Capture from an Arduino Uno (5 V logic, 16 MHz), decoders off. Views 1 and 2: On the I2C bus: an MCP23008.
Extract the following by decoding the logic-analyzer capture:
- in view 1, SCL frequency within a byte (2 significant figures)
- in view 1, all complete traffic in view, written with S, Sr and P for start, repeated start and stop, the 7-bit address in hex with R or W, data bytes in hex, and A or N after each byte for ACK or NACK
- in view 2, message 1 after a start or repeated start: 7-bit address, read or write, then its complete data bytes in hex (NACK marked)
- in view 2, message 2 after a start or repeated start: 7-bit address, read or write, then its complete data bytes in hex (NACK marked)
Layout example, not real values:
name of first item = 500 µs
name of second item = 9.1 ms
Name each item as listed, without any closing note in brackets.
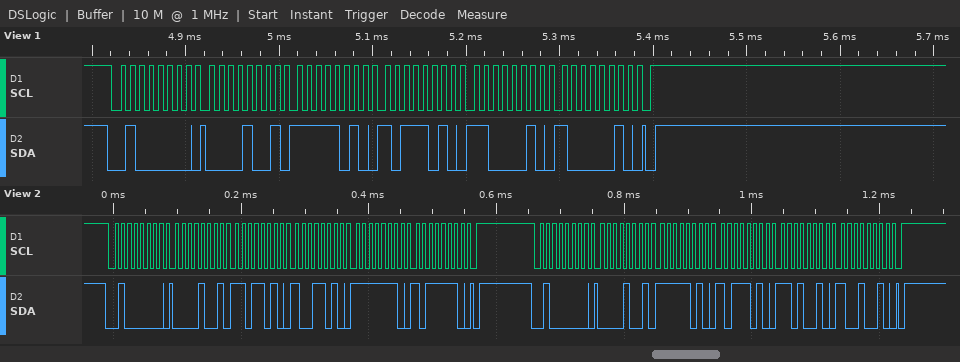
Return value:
in view 1, SCL frequency within a byte = 100 kHz
in view 1, all complete traffic in view, written with S, Sr and P for start, repeated start and stop, the 7-bit address in hex with R or W, data bytes in hex, and A or N after each byte for ACK or NACK = S 20W A 09 A FA A BA A C2 A 82 A P
in view 2, message 1 after a start or repeated start: 7-bit address, read or write, then its complete data bytes in hex = 0x20 write: 09 DA 9A FE BE
in view 2, message 2 after a start or repeated start: 7-bit address, read or write, then its complete data bytes in hex = 0x20 write: 09 FA BA D2 92
